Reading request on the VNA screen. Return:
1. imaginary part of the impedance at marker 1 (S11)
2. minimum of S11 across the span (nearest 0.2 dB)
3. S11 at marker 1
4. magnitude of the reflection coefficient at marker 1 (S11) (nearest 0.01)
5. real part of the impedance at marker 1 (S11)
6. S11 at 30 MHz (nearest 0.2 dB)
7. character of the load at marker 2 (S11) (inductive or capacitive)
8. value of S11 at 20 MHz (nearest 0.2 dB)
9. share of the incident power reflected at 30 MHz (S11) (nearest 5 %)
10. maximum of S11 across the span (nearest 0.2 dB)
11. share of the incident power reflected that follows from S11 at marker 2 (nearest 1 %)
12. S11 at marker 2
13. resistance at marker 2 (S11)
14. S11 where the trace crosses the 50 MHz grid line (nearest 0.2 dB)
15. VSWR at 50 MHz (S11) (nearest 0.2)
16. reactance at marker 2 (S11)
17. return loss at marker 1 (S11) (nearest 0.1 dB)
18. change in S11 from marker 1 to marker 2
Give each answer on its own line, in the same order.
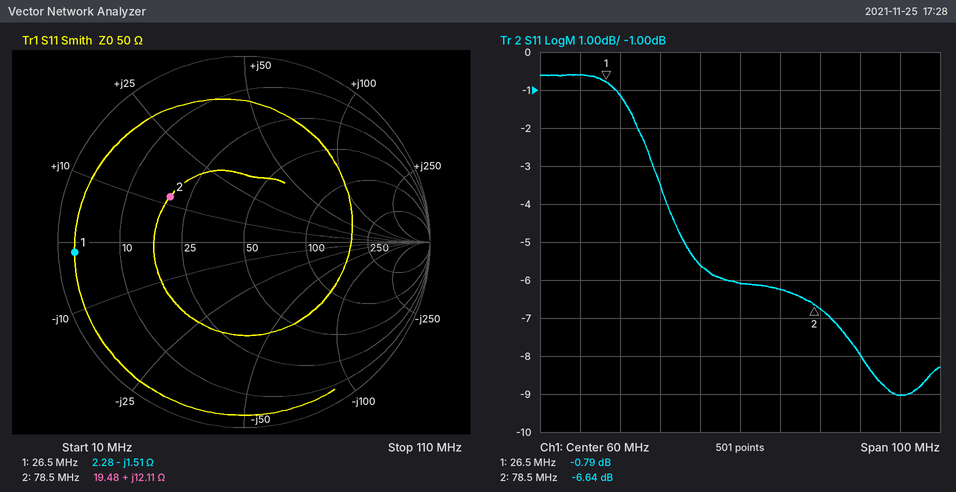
-1.51 Ω
-9.0 dB
-0.79 dB
0.91
2.28 Ω
-1.2 dB
inductive
-0.6 dB
75 %
-0.6 dB
22 %
-6.64 dB
19.48 Ω
-5.6 dB
3.2
+12.11 Ω
0.8 dB
-5.85 dB
